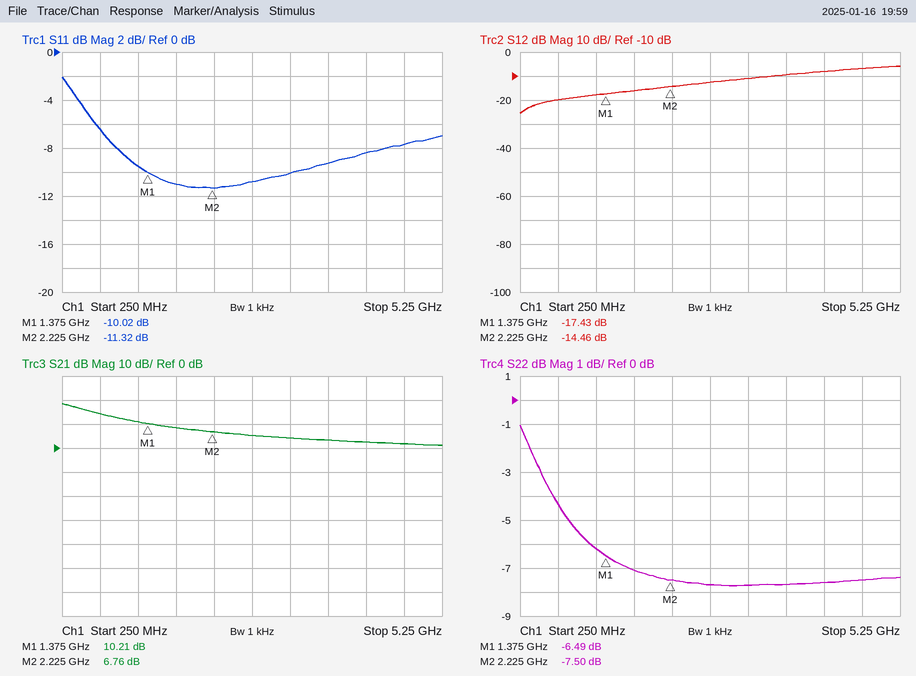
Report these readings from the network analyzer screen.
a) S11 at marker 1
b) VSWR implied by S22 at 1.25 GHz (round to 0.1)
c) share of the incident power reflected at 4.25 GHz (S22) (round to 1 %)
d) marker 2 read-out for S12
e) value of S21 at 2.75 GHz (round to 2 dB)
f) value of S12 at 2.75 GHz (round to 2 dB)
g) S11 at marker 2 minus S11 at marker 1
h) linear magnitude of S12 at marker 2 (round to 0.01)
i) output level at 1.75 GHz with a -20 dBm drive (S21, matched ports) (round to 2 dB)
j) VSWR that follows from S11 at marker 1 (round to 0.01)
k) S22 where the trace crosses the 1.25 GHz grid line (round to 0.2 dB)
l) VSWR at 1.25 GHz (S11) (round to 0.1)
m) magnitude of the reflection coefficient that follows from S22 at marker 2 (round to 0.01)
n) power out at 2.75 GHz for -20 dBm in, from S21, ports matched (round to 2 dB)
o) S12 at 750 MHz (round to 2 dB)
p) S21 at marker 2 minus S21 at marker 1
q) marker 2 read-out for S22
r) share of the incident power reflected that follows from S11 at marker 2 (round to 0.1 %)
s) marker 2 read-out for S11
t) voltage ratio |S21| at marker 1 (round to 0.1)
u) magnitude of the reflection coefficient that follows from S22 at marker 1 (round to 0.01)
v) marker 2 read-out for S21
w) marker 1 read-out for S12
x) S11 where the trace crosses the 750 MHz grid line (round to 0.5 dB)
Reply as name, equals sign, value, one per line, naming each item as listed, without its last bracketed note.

S11 at marker 1 = -10.02 dB
VSWR implied by S22 at 1.25 GHz = 2.9
share of the incident power reflected at 4.25 GHz (S22) = 17 %
marker 2 read-out for S12 = -14.46 dB
value of S21 at 2.75 GHz = 6 dB
value of S12 at 2.75 GHz = -12 dB
S11 at marker 2 minus S11 at marker 1 = -1.30 dB
linear magnitude of S12 at marker 2 = 0.19
output level at 1.75 GHz with a -20 dBm drive (S21, matched ports) = -12 dBm
VSWR that follows from S11 at marker 1 = 1.92
S22 where the trace crosses the 1.25 GHz grid line = -6.2 dB
VSWR at 1.25 GHz (S11) = 2.0
magnitude of the reflection coefficient that follows from S22 at marker 2 = 0.42
power out at 2.75 GHz for -20 dBm in, from S21, ports matched = -14 dBm
S12 at 750 MHz = -20 dB
S21 at marker 2 minus S21 at marker 1 = -3.45 dB
marker 2 read-out for S22 = -7.50 dB
share of the incident power reflected that follows from S11 at marker 2 = 7.4 %
marker 2 read-out for S11 = -11.32 dB
voltage ratio |S21| at marker 1 = 3.2
magnitude of the reflection coefficient that follows from S22 at marker 1 = 0.47
marker 2 read-out for S21 = 6.76 dB
marker 1 read-out for S12 = -17.43 dB
S11 where the trace crosses the 750 MHz grid line = -6.5 dB
